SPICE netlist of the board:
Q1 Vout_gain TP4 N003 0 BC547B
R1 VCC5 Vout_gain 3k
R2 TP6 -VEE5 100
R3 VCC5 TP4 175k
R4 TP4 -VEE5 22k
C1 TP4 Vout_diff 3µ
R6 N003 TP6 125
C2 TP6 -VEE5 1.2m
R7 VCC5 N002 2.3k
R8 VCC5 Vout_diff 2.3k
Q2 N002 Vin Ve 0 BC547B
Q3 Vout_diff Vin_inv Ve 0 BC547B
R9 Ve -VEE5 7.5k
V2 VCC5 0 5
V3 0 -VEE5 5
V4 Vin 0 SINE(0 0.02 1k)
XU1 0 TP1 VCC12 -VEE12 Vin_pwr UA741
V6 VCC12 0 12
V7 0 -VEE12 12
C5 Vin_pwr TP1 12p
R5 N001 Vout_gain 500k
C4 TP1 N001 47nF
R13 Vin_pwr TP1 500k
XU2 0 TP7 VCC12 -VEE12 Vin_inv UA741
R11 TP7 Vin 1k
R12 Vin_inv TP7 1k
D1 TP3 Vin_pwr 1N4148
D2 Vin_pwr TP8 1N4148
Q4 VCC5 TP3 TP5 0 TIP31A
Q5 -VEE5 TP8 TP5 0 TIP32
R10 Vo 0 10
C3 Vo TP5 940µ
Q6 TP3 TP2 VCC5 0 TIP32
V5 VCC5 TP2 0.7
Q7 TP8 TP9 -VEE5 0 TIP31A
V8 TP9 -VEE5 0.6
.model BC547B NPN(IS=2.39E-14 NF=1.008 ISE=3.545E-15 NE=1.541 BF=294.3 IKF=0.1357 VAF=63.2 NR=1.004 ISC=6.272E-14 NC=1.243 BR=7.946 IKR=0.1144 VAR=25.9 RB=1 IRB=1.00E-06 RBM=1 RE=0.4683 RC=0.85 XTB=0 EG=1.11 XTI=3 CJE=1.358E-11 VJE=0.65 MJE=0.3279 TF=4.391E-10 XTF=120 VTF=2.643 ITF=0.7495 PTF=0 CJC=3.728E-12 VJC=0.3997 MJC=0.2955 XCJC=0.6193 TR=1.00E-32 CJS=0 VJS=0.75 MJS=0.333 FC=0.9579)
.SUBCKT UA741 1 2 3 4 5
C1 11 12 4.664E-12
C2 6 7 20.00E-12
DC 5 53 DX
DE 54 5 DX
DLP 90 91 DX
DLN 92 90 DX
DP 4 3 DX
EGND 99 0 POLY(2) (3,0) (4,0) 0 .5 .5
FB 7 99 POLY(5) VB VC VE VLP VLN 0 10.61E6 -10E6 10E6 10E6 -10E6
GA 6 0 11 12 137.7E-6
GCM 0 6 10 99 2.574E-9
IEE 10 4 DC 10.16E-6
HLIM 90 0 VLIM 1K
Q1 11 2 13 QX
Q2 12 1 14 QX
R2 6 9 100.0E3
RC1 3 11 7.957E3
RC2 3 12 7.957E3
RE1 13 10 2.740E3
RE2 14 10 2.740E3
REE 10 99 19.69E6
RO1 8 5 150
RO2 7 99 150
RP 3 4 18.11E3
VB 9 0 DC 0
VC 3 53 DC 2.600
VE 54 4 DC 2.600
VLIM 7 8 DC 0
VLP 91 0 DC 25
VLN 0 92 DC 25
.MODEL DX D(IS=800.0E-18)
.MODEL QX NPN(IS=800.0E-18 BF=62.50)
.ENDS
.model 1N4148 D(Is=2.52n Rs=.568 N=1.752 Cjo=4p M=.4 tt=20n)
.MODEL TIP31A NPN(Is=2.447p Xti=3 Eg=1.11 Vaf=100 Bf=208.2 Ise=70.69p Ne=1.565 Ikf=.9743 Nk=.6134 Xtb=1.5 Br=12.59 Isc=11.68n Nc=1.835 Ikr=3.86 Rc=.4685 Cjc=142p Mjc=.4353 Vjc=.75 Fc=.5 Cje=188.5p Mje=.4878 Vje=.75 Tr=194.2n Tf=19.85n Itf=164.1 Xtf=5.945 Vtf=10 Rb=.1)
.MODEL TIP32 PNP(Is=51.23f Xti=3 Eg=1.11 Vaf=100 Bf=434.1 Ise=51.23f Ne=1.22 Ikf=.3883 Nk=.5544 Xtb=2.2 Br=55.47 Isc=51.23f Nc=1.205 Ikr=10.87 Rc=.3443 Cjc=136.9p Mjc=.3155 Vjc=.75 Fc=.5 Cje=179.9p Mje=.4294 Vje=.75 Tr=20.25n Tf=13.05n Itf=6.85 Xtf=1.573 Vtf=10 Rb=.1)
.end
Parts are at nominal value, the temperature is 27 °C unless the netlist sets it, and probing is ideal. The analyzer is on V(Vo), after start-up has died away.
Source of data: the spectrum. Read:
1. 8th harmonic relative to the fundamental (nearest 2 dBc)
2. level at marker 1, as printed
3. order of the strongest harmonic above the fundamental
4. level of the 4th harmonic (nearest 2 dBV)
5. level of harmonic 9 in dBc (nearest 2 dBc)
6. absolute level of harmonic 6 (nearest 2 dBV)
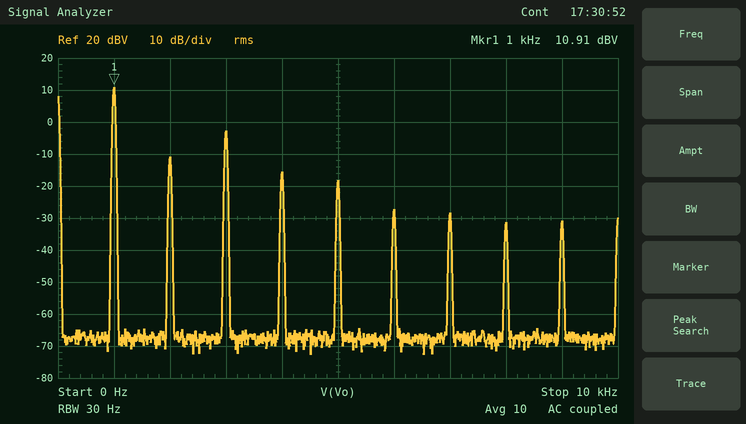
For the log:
-42 dBc
10.91 dBV
3
-16 dBV
-42 dBc
-28 dBV
